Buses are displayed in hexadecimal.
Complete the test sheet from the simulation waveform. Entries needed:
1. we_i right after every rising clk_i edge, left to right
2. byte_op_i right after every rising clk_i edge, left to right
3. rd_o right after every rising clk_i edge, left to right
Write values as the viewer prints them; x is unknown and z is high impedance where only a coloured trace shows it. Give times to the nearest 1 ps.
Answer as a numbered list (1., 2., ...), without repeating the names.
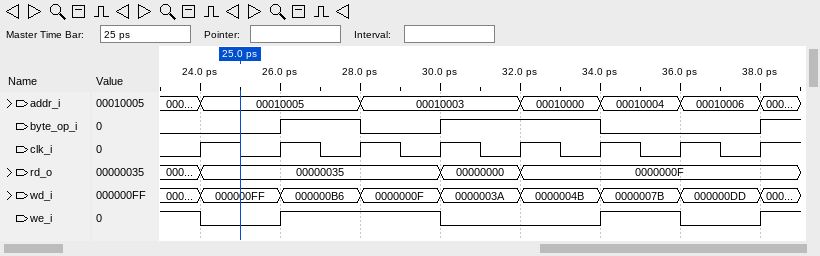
1. 0 1 1 0 0 1 0 1
2. 0 1 0 1 1 0 0 1
3. 00000035, 00000035, 00000035, 00000000, 0000000F, 0000000F, 0000000F, 0000000F
